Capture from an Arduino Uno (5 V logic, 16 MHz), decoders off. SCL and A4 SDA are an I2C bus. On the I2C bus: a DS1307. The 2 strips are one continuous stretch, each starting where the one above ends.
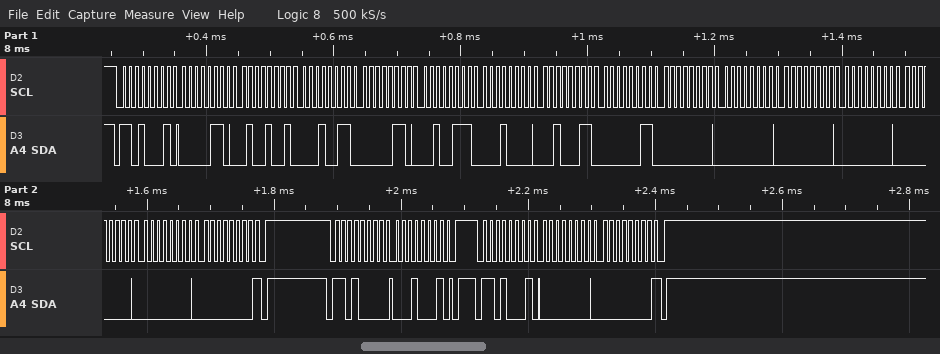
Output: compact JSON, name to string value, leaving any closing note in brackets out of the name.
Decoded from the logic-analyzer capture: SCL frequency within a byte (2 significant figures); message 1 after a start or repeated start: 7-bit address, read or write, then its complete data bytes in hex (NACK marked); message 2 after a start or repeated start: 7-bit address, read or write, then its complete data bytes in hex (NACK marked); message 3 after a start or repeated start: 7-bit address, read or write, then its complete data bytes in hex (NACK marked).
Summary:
{"SCL frequency within a byte": "100 kHz", "message 1 after a start or repeated start: 7-bit address, read or write, then its complete data bytes in hex": "0x68 read: 06 49 13 06 27 10 23 03 00 00 00 00 00 00 00 NACK", "message 2 after a start or repeated start: 7-bit address, read or write, then its complete data bytes in hex": "0x68 write: 11", "message 3 after a start or repeated start: 7-bit address, read or write, then its complete data bytes in hex": "0x68 read: 00 00 NACK"}
